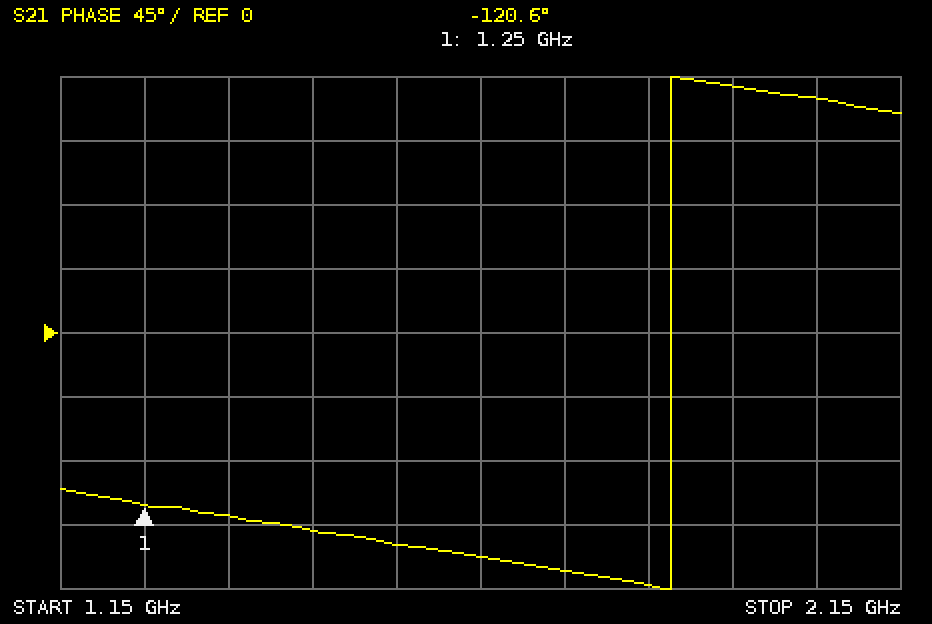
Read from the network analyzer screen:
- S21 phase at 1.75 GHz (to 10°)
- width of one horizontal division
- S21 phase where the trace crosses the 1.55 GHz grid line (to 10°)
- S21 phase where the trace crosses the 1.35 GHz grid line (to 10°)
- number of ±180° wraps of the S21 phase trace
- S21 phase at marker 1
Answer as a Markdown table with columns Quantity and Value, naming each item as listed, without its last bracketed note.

| Quantity | Value |
|---|---|
| S21 phase at 1.75 GHz | -170° |
| width of one horizontal division | 100 MHz |
| S21 phase where the trace crosses the 1.55 GHz grid line | -150° |
| S21 phase where the trace crosses the 1.35 GHz grid line | -130° |
| number of ±180° wraps of the S21 phase trace | 1 |
| S21 phase at marker 1 | -120.6° |
